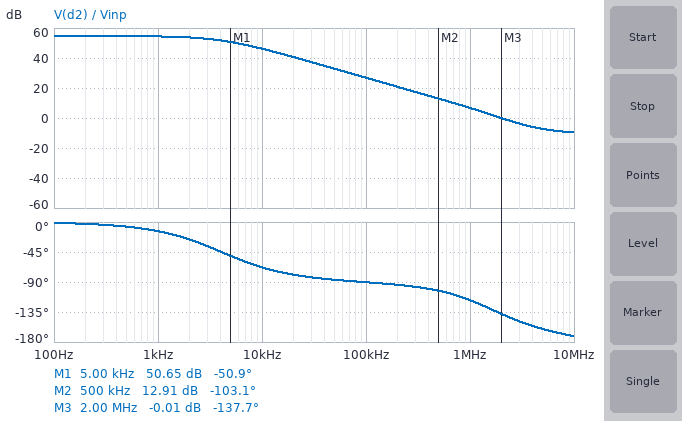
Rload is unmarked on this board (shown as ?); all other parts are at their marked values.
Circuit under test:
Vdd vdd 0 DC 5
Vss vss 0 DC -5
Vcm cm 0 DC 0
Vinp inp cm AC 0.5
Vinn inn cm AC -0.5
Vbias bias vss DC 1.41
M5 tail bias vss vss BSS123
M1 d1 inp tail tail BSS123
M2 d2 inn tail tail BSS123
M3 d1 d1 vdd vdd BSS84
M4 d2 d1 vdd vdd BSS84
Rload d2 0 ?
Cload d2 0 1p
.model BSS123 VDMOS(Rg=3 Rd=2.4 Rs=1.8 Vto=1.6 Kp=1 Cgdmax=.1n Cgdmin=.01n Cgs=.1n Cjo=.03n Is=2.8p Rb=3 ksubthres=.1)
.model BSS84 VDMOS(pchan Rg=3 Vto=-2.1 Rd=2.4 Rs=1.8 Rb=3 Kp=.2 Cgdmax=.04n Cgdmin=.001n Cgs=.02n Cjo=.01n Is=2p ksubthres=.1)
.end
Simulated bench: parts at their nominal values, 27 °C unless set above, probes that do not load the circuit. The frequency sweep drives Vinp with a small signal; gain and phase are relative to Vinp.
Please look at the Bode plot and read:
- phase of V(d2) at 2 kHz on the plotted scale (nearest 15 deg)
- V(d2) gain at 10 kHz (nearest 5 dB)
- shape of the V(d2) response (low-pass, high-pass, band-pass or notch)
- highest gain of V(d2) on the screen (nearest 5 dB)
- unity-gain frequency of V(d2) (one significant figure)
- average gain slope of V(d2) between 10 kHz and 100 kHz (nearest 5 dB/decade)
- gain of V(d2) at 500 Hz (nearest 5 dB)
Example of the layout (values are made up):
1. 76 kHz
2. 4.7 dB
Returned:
1. -30 deg
2. 45 dB
3. low-pass
4. 55 dB
5. 2 MHz
6. -20 dB/decade
7. 55 dB
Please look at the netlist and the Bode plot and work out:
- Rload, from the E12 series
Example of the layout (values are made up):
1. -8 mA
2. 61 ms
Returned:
1. 390 kΩ
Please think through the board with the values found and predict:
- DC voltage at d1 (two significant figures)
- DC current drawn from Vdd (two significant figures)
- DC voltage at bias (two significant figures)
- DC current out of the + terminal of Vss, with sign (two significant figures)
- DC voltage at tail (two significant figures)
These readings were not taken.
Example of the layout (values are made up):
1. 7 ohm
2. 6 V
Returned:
1. 3.0 V
2. 97 µA
3. -3.6 V
4. -97 µA
5. -1.4 V
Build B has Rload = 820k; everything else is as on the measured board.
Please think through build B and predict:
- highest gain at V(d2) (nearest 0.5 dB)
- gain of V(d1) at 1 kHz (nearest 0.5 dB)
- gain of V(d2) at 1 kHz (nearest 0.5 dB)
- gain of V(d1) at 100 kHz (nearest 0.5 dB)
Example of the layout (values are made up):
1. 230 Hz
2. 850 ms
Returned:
1. 61.0 dB
2. -2.5 dB
3. 60.0 dB
4. -5.0 dB
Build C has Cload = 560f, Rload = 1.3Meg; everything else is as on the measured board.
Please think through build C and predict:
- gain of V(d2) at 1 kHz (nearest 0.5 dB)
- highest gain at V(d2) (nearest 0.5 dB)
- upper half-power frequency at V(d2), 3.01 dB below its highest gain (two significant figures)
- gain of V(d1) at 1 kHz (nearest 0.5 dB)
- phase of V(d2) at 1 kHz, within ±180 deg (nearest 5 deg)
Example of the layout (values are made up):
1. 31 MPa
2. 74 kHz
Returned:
1. 63.0 dB
2. 65.0 dB
3. 1.2 kHz
4. -3.0 dB
5. -40 deg
